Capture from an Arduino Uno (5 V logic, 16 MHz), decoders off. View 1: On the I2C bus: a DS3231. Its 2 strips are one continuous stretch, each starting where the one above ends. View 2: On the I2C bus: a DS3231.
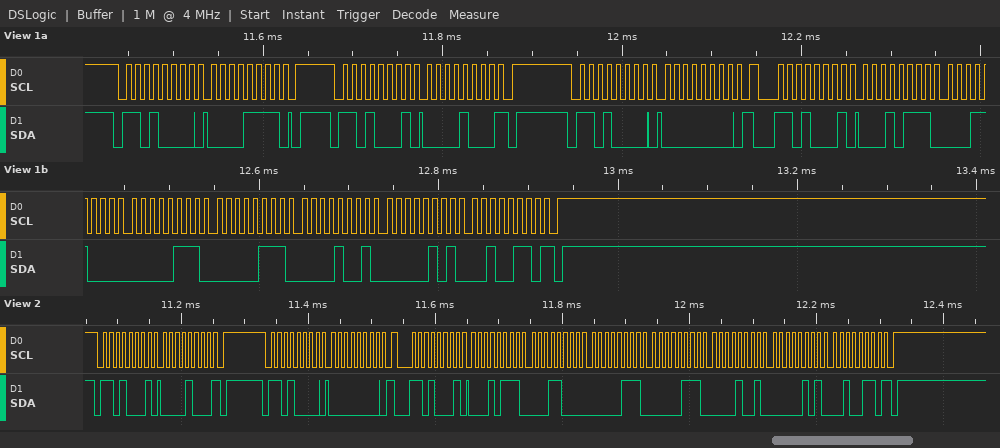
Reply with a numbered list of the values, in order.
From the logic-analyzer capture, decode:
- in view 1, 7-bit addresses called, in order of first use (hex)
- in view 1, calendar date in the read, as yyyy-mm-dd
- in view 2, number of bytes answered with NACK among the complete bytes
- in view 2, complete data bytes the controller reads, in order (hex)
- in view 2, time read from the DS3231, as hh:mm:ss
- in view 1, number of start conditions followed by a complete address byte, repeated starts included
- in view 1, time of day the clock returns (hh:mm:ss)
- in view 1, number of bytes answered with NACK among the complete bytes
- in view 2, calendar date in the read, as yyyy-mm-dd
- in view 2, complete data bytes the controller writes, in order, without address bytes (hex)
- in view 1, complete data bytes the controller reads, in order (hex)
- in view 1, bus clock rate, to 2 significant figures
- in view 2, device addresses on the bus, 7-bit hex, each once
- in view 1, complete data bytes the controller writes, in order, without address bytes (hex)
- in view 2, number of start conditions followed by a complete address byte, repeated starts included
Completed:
1. 0x68
2. 2026-05-09
3. 2
4. 08 17 18 07 07 09 05 26
5. 07:18:17
6. 4
7. 07:18:17
8. 2
9. 2026-05-09
10. 00
11. 08 17 18 07 07 09 05 26
12. 100 kHz
13. 0x68
14. 0F 00
15. 3
